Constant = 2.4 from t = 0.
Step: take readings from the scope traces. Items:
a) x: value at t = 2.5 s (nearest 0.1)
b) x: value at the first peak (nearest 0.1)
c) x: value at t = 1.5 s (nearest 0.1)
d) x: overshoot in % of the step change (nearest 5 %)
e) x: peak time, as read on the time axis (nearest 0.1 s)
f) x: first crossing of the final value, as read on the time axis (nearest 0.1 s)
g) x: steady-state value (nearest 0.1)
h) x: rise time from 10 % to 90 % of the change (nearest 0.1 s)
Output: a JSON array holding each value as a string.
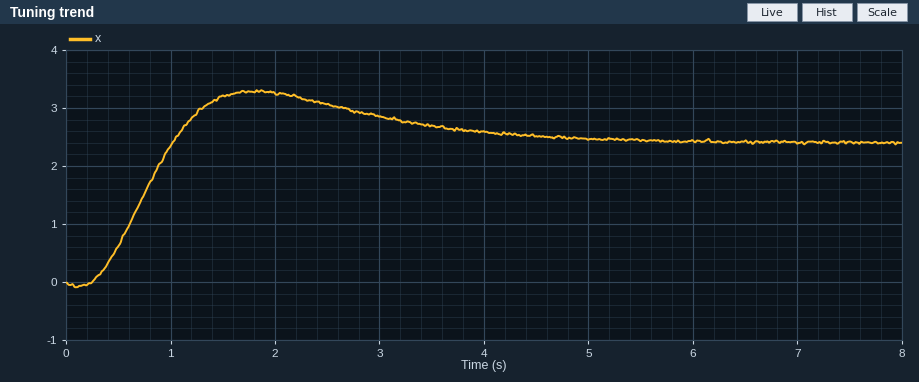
["3.1", "3.3", "3.2", "35 %", "1.8 s", "1.0 s", "2.4", "0.6 s"]
